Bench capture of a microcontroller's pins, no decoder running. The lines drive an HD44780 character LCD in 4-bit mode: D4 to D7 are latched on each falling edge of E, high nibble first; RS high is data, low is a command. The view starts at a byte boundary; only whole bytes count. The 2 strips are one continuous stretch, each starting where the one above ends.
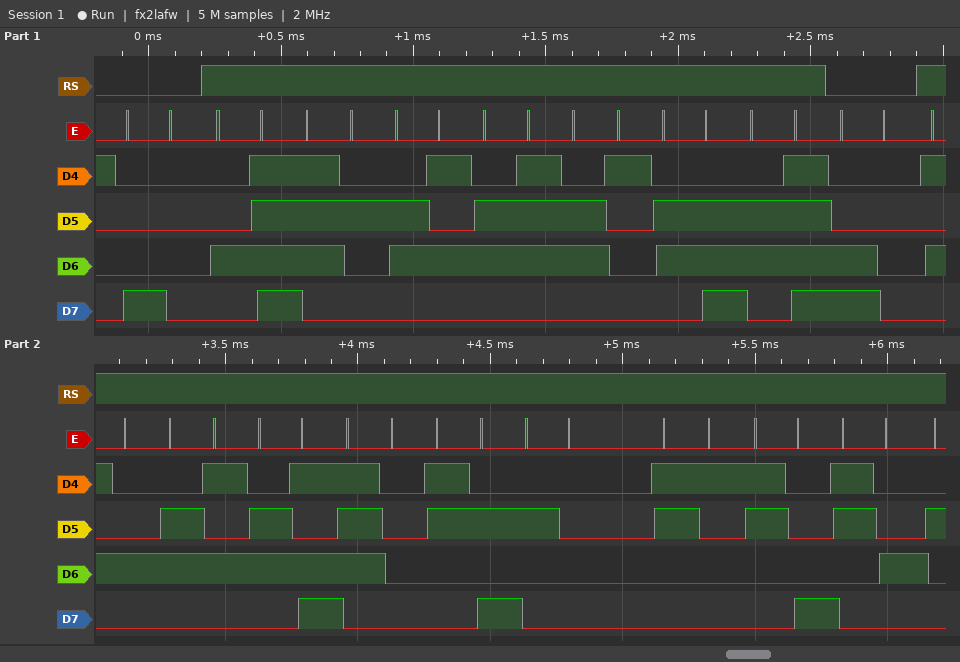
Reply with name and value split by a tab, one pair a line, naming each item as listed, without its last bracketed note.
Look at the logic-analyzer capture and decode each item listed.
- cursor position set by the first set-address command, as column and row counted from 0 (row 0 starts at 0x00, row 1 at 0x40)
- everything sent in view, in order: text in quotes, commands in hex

cursor position set by the first set-address command, as column and row counted from 0	column 0, row 0
everything sent in view, in order: text in quotes, commands in hex	0x80 "Oregano" 0xC0 "Temp: 184"
